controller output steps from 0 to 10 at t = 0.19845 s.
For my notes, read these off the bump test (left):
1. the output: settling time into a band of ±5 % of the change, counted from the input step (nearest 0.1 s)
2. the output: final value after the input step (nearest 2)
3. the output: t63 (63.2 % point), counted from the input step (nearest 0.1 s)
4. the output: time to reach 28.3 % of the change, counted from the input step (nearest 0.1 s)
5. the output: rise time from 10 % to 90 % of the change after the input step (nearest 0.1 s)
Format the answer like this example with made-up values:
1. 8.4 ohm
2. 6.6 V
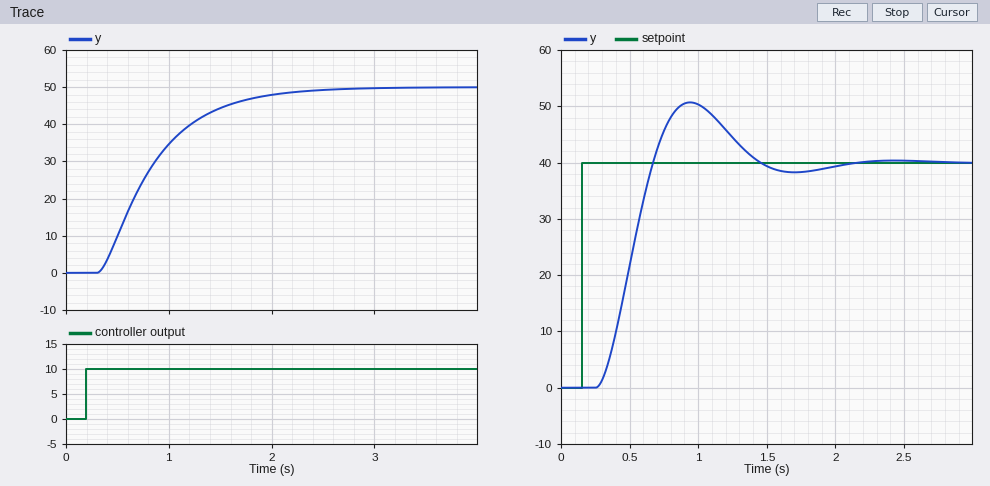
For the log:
1. 1.7 s
2. 50
3. 0.7 s
4. 0.4 s
5. 1.1 s
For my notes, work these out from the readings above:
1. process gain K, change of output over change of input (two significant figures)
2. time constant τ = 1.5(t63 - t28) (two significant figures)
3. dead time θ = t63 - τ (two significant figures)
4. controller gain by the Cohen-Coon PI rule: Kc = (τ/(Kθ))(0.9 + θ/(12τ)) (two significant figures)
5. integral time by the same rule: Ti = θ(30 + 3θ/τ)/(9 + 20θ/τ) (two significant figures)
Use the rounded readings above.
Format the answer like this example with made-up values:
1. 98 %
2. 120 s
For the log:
1. 5.0
2. 0.45 s
3. 0.25 s
4. 0.34
5. 0.39 s
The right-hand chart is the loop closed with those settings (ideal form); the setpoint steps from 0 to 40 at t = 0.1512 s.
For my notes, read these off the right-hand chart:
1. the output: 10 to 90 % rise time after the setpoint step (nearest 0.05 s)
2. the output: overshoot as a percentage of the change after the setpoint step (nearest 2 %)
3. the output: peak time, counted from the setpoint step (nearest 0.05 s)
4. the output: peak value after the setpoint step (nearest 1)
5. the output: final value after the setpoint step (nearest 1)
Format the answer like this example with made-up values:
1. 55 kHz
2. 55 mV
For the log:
1. 0.30 s
2. 26 %
3. 0.80 s
4. 51
5. 40
